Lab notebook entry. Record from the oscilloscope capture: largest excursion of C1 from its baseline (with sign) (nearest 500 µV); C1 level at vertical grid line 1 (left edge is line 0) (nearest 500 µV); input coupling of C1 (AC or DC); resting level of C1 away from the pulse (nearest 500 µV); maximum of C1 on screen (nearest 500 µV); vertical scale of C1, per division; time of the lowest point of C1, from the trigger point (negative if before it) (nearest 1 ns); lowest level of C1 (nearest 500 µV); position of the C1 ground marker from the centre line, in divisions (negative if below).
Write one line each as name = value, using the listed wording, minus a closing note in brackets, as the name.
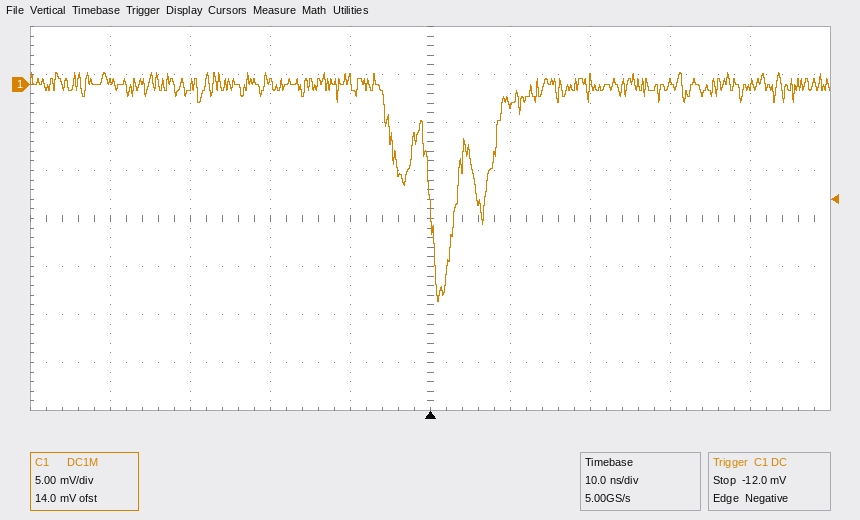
largest excursion of C1 from its baseline (with sign) = -22.5 mV
C1 level at vertical grid line 1 (left edge is line 0) = 500 µV
input coupling of C1 = DC
resting level of C1 away from the pulse = 0.0 mV
maximum of C1 on screen = 1.0 mV
vertical scale of C1, per division = 5 mV
time of the lowest point of C1, from the trigger point (negative if before it) = +1 ns
lowest level of C1 = -22.5 mV
position of the C1 ground marker from the centre line, in divisions = +2.8 div
